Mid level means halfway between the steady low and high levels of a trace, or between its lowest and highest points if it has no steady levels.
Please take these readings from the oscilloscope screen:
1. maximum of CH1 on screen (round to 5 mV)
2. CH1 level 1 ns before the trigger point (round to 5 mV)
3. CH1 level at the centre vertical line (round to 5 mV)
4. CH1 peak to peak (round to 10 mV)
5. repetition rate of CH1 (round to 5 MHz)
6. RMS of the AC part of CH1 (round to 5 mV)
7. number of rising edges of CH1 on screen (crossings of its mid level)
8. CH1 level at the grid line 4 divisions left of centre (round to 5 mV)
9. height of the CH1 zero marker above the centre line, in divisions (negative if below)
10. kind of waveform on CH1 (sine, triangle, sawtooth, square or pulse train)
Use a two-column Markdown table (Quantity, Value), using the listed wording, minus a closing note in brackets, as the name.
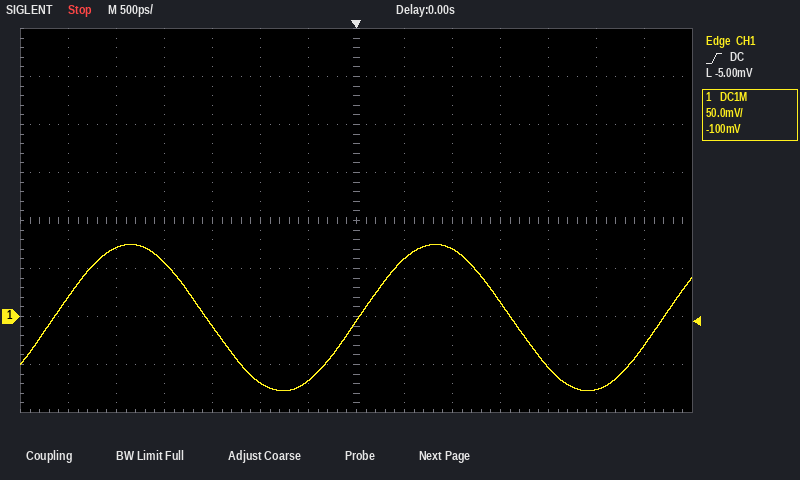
| Quantity | Value |
|---|---|
| maximum of CH1 on screen | 75 mV |
| CH1 level 1 ns before the trigger point | -70 mV |
| CH1 level at the centre vertical line | -5 mV |
| CH1 peak to peak | 150 mV |
| repetition rate of CH1 | 315 MHz |
| RMS of the AC part of CH1 | 55 mV |
| number of rising edges of CH1 on screen | 3 |
| CH1 level at the grid line 4 divisions left of centre | 55 mV |
| height of the CH1 zero marker above the centre line, in divisions | -2.0 div |
| kind of waveform on CH1 | sine |
